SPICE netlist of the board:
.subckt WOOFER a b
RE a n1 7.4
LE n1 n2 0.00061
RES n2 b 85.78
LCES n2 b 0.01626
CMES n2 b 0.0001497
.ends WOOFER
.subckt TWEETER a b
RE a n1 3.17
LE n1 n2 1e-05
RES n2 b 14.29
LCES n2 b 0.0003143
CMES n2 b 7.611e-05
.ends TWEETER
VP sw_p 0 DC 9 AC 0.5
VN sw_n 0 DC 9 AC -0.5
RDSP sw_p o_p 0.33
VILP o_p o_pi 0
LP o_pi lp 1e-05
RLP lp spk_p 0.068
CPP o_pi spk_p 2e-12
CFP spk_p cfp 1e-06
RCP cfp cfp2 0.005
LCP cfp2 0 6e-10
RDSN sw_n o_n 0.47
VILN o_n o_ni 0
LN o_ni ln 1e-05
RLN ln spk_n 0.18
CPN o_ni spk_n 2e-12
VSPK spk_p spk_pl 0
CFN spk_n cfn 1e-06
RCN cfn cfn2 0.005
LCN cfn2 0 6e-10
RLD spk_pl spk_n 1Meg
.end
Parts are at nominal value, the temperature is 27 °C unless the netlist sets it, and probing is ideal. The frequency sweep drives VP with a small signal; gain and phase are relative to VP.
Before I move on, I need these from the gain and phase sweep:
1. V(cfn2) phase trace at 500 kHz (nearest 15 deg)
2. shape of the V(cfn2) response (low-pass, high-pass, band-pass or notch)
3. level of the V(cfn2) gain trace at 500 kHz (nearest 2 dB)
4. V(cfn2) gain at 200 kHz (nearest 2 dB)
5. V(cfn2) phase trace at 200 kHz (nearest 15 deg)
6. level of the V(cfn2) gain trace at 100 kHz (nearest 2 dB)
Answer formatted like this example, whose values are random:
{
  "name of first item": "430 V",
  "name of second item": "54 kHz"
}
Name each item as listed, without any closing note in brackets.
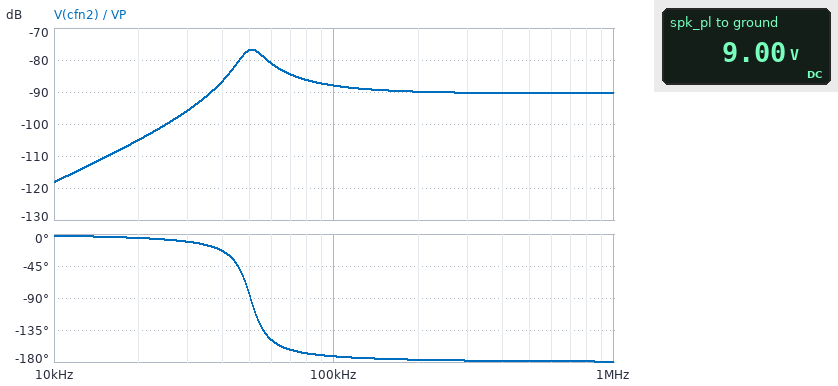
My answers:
{
  "V(cfn2) phase trace at 500 kHz": "-180 deg",
  "shape of the V(cfn2) response": "high-pass",
  "level of the V(cfn2) gain trace at 500 kHz": "-90 dB",
  "V(cfn2) gain at 200 kHz": "-90 dB",
  "V(cfn2) phase trace at 200 kHz": "-180 deg",
  "level of the V(cfn2) gain trace at 100 kHz": "-88 dB"
}
